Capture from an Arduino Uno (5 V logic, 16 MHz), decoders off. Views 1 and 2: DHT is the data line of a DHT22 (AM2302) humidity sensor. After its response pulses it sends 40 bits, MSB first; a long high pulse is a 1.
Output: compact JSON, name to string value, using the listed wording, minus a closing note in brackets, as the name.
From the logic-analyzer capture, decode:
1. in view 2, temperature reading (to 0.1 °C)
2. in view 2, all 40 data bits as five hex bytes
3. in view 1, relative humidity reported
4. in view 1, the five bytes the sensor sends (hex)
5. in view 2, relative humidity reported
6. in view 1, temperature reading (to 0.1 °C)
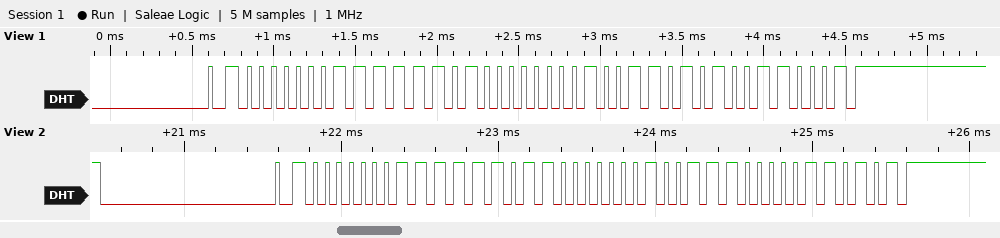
{"in view 2, temperature reading": "31.2 °C", "in view 2, all 40 data bits as five hex bytes": "01 FB 01 38 35", "in view 1, relative humidity reported": "50.6 %", "in view 1, the five bytes the sensor sends": "01 FA 01 35 31", "in view 2, relative humidity reported": "50.7 %", "in view 1, temperature reading": "30.9 °C"}
